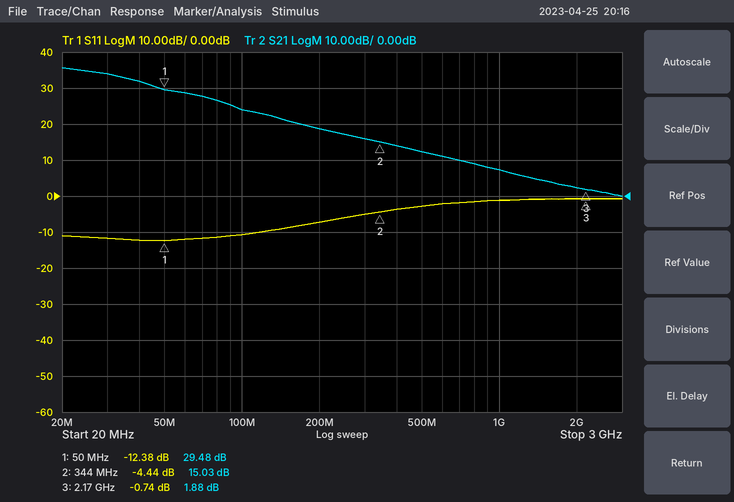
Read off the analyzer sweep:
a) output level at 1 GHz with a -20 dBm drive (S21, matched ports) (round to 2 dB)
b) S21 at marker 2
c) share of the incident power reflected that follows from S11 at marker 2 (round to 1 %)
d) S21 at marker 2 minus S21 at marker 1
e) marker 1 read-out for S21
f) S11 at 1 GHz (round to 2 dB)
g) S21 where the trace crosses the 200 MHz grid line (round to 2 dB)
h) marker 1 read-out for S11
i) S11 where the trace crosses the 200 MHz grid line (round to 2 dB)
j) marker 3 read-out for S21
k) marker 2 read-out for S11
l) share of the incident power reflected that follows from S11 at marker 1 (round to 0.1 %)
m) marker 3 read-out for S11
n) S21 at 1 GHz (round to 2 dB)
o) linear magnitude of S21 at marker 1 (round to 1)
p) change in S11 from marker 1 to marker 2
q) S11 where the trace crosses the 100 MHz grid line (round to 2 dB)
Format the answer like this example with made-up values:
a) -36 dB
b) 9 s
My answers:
a) -12 dBm
b) 15.03 dB
c) 36 %
d) -14.45 dB
e) 29.48 dB
f) -2 dB
g) 18 dB
h) -12.38 dB
i) -8 dB
j) 1.88 dB
k) -4.44 dB
l) 5.8 %
m) -0.74 dB
n) 8 dB
o) 30
p) 7.94 dB
q) -10 dB
